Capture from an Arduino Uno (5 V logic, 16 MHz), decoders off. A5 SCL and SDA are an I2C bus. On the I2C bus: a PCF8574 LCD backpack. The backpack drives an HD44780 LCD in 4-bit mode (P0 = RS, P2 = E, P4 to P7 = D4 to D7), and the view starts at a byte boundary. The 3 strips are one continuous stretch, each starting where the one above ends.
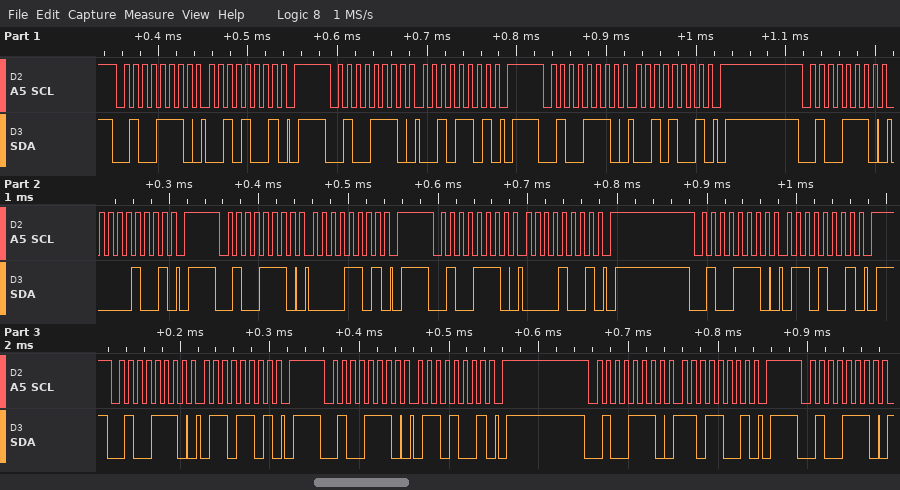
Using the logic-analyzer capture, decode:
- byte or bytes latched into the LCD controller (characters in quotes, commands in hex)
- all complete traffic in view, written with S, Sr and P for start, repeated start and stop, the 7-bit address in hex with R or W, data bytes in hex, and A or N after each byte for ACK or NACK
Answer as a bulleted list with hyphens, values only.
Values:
- ' '
- S 27W A 29 A P S 27W A 2D A P S 27W A 29 A P S 27W A 09 A P S 27W A 0D A P S 27W A 09 A P S 27W A 69 A P S 27W A 6D A P S 27W A 69 A P S 27W A D9 A P S 27W A
